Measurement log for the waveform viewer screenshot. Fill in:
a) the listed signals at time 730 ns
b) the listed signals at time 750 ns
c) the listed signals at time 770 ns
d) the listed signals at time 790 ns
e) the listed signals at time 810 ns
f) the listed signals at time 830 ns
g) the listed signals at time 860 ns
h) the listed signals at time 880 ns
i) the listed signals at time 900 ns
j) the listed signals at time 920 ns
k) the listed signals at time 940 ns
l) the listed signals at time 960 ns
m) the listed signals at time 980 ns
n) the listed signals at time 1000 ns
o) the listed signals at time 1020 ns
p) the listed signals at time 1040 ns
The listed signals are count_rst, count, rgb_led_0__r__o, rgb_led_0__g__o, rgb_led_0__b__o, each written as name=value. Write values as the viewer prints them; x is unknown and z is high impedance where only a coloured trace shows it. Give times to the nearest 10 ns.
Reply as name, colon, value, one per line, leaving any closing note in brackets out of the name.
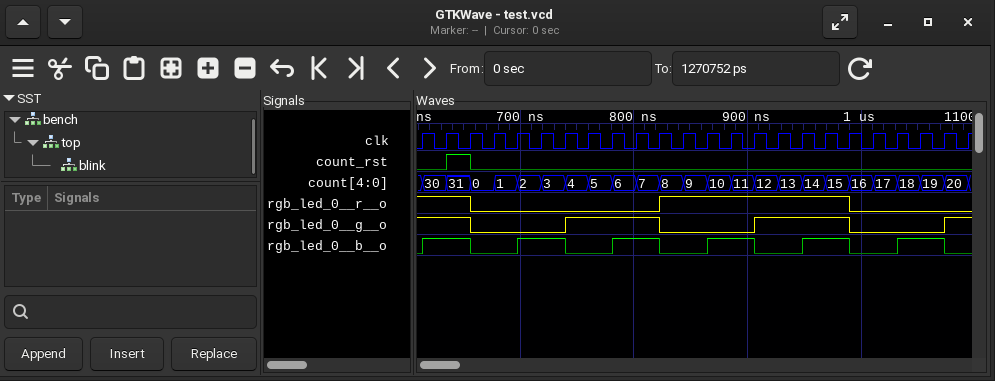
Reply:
the listed signals at time 730 ns: count_rst=0, count=3, rgb_led_0__r__o=0, rgb_led_0__g__o=0, rgb_led_0__b__o=1
the listed signals at time 750 ns: count_rst=0, count=4, rgb_led_0__r__o=0, rgb_led_0__g__o=1, rgb_led_0__b__o=0
the listed signals at time 770 ns: count_rst=0, count=5, rgb_led_0__r__o=0, rgb_led_0__g__o=1, rgb_led_0__b__o=0
the listed signals at time 790 ns: count_rst=0, count=6, rgb_led_0__r__o=0, rgb_led_0__g__o=1, rgb_led_0__b__o=1
the listed signals at time 810 ns: count_rst=0, count=7, rgb_led_0__r__o=0, rgb_led_0__g__o=1, rgb_led_0__b__o=1
the listed signals at time 830 ns: count_rst=0, count=8, rgb_led_0__r__o=1, rgb_led_0__g__o=0, rgb_led_0__b__o=0
the listed signals at time 860 ns: count_rst=0, count=9, rgb_led_0__r__o=1, rgb_led_0__g__o=0, rgb_led_0__b__o=0
the listed signals at time 880 ns: count_rst=0, count=10, rgb_led_0__r__o=1, rgb_led_0__g__o=0, rgb_led_0__b__o=1
the listed signals at time 900 ns: count_rst=0, count=11, rgb_led_0__r__o=1, rgb_led_0__g__o=0, rgb_led_0__b__o=1
the listed signals at time 920 ns: count_rst=0, count=12, rgb_led_0__r__o=1, rgb_led_0__g__o=1, rgb_led_0__b__o=0
the listed signals at time 940 ns: count_rst=0, count=13, rgb_led_0__r__o=1, rgb_led_0__g__o=1, rgb_led_0__b__o=0
the listed signals at time 960 ns: count_rst=0, count=14, rgb_led_0__r__o=1, rgb_led_0__g__o=1, rgb_led_0__b__o=1
the listed signals at time 980 ns: count_rst=0, count=15, rgb_led_0__r__o=1, rgb_led_0__g__o=1, rgb_led_0__b__o=1
the listed signals at time 1000 ns: count_rst=0, count=16, rgb_led_0__r__o=0, rgb_led_0__g__o=0, rgb_led_0__b__o=0
the listed signals at time 1020 ns: count_rst=0, count=17, rgb_led_0__r__o=0, rgb_led_0__g__o=0, rgb_led_0__b__o=0
the listed signals at time 1040 ns: count_rst=0, count=18, rgb_led_0__r__o=0, rgb_led_0__g__o=0, rgb_led_0__b__o=1
